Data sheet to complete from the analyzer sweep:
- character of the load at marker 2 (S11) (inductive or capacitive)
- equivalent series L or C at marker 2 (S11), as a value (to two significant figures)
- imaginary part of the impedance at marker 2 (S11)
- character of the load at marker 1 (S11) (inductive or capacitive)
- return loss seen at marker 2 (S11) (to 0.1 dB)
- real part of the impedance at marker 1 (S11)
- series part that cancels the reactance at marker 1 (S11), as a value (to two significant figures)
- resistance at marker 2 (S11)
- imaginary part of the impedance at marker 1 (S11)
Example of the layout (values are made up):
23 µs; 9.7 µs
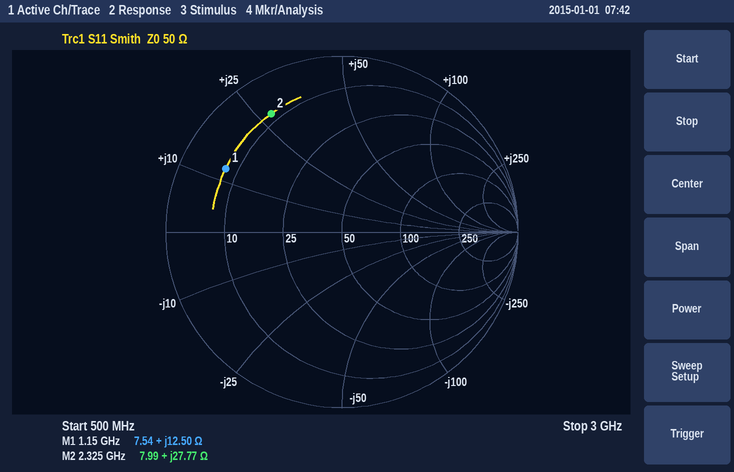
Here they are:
inductive; 1.9 nH; +27.77 Ω; inductive; 2.1 dB; 7.54 Ω; 11 pF; 7.99 Ω; +12.50 Ω
